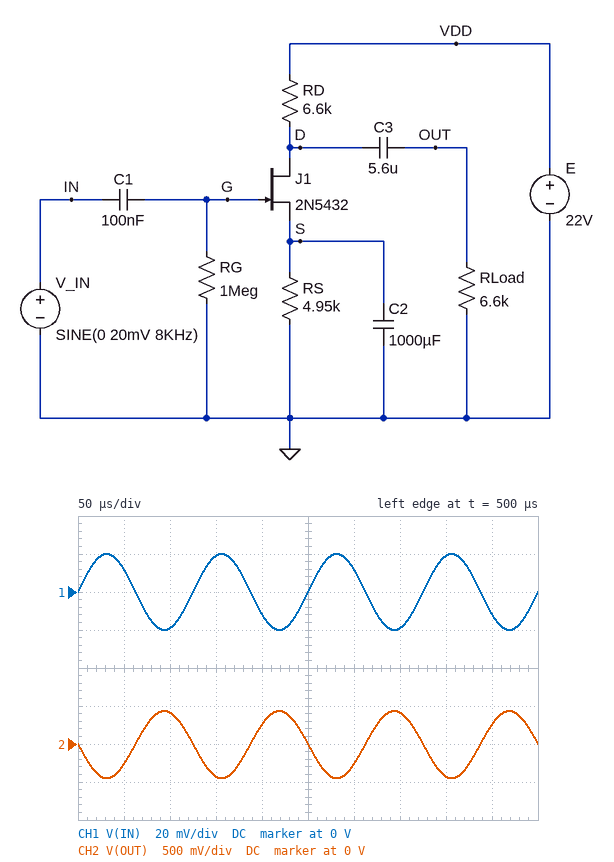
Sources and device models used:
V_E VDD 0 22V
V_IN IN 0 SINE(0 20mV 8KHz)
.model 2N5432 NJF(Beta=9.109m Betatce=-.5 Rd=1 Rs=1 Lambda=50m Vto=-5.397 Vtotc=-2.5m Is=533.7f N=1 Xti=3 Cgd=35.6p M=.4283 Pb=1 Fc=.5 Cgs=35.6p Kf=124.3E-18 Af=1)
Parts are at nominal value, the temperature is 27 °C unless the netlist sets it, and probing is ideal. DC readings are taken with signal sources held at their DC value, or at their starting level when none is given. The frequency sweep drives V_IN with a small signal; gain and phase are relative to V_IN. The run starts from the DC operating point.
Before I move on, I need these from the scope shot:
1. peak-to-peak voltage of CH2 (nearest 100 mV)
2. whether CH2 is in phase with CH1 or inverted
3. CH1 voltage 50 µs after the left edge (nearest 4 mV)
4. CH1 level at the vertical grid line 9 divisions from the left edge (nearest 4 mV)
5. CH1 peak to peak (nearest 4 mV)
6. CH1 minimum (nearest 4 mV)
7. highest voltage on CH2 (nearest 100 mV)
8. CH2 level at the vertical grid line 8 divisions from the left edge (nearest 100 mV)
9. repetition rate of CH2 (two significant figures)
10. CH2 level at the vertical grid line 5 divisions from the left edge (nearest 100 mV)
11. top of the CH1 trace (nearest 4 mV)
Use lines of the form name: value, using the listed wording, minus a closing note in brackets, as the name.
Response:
peak-to-peak voltage of CH2: 900 mV
whether CH2 is in phase with CH1 or inverted: inverted
CH1 voltage 50 µs after the left edge: 12 mV
CH1 level at the vertical grid line 9 divisions from the left edge: -12 mV
CH1 peak to peak: 40 mV
CH1 minimum: -20 mV
highest voltage on CH2: 400 mV
CH2 level at the vertical grid line 8 divisions from the left edge: -400 mV
repetition rate of CH2: 8.0 kHz
CH2 level at the vertical grid line 5 divisions from the left edge: 0 V
top of the CH1 trace: 20 mV
